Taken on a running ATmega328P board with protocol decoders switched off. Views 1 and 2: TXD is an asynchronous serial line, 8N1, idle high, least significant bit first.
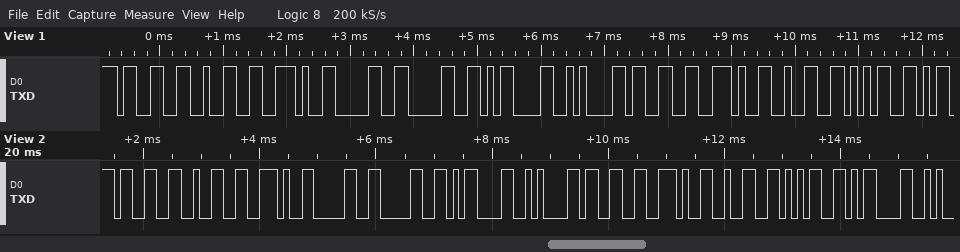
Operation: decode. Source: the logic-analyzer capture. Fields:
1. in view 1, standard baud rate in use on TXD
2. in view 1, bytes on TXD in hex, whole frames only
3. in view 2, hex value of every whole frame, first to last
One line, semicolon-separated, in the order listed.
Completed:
9600 baud; 33 32 2E 30 30 0D 0A 33 2E 32 35; 33 32 2E 30 30 0D 0A 33 2E 32 35 0D
